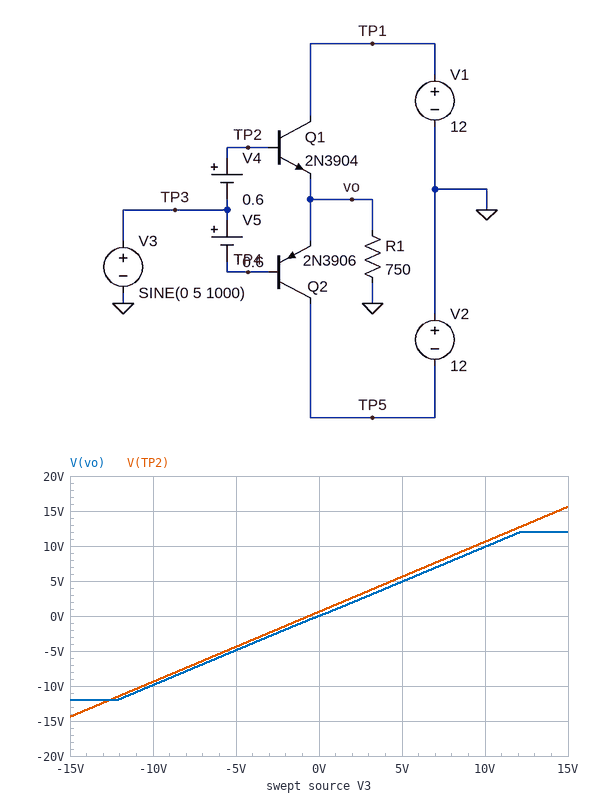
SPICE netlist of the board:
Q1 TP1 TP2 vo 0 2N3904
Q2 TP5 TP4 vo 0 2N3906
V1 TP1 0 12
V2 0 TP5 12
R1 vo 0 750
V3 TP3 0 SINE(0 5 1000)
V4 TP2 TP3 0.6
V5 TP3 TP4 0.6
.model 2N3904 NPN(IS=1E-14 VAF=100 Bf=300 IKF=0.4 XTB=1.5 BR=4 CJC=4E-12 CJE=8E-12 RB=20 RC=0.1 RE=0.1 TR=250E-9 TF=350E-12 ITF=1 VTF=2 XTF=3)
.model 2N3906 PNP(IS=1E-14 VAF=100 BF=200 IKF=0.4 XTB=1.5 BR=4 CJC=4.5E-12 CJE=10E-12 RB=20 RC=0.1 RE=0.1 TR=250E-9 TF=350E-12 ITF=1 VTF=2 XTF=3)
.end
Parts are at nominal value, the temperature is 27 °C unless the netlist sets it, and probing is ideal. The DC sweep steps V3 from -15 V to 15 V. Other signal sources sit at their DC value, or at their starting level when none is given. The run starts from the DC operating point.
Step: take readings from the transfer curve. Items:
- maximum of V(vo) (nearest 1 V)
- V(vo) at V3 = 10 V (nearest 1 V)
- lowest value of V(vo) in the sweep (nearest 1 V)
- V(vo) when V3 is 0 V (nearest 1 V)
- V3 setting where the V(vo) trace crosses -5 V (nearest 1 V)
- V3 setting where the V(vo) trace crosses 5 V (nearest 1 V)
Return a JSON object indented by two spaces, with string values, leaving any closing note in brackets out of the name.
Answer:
{
  "maximum of V(vo)": "12 V",
  "V(vo) at V3 = 10 V": "10 V",
  "lowest value of V(vo) in the sweep": "-12 V",
  "V(vo) when V3 is 0 V": "0 V",
  "V3 setting where the V(vo) trace crosses -5 V": "-5 V",
  "V3 setting where the V(vo) trace crosses 5 V": "5 V"
}
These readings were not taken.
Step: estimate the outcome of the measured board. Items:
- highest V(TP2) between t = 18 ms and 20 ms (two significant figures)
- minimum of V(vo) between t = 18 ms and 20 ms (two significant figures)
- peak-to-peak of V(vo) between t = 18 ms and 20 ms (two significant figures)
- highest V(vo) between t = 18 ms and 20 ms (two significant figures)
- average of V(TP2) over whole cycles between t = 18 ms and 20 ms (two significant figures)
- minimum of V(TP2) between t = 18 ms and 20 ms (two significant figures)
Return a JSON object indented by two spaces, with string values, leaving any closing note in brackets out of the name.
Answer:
{
  "highest V(TP2) between t = 18 ms and 20 ms": "5.6 V",
  "minimum of V(vo) between t = 18 ms and 20 ms": "-4.9 V",
  "peak-to-peak of V(vo) between t = 18 ms and 20 ms": "9.8 V",
  "highest V(vo) between t = 18 ms and 20 ms": "4.9 V",
  "average of V(TP2) over whole cycles between t = 18 ms and 20 ms": "600 mV",
  "minimum of V(TP2) between t = 18 ms and 20 ms": "-4.4 V"
}
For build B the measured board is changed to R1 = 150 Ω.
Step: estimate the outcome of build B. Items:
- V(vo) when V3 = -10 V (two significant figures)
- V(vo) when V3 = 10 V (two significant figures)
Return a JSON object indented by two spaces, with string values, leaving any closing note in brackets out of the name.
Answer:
{
  "V(vo) when V3 = -10 V": "-9.8 V",
  "V(vo) when V3 = 10 V": "9.8 V"
}
